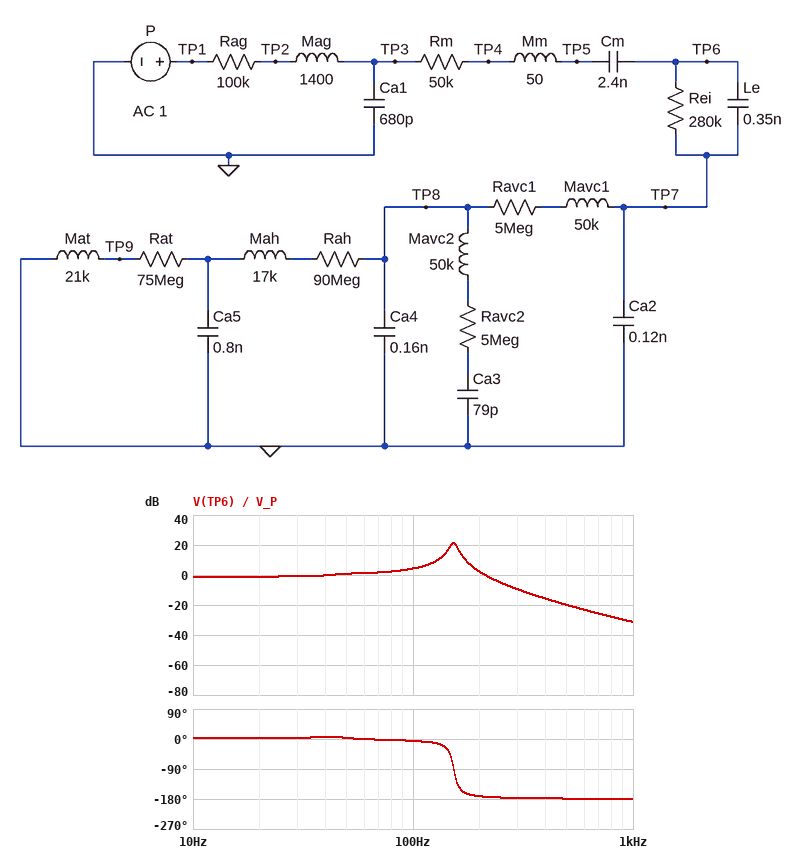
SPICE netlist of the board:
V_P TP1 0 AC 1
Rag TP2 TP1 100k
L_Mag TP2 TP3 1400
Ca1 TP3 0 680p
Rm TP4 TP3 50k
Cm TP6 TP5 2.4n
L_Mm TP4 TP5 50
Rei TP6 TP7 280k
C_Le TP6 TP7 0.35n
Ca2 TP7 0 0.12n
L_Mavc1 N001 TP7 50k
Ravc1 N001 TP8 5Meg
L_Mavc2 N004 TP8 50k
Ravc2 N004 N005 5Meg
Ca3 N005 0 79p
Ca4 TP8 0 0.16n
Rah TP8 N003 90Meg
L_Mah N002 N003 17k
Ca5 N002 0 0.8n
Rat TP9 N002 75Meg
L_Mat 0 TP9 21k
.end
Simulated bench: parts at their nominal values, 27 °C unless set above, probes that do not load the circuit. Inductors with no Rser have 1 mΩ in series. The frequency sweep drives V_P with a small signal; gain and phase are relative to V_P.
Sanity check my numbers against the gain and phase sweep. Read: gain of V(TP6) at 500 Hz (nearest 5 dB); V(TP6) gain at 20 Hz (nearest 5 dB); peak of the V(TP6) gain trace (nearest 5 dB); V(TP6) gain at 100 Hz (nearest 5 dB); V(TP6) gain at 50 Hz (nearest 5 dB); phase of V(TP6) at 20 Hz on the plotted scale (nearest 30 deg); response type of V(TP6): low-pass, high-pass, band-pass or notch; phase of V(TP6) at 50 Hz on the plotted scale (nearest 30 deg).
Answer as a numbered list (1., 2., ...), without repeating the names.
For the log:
1. -20 dB
2. 0 dB
3. 20 dB
4. 5 dB
5. 0 dB
6. 0 deg
7. low-pass
8. 0 deg
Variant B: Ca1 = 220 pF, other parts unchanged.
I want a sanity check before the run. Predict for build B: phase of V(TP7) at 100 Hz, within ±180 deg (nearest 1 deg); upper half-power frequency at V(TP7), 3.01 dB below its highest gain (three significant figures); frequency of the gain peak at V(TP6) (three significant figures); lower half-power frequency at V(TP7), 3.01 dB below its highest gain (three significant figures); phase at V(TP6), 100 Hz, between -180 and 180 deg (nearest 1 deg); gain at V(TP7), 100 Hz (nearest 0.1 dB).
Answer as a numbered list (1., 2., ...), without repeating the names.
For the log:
1. -3 deg
2. 243 Hz
3. 235 Hz
4. 228 Hz
5. -2 deg
6. 1.2 dB
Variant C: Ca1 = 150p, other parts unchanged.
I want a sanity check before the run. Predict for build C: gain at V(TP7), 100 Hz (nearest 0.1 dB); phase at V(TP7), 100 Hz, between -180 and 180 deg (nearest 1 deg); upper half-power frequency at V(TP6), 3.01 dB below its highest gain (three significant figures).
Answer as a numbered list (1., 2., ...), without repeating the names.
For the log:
1. 0.8 dB
2. -2 deg
3. 273 Hz
